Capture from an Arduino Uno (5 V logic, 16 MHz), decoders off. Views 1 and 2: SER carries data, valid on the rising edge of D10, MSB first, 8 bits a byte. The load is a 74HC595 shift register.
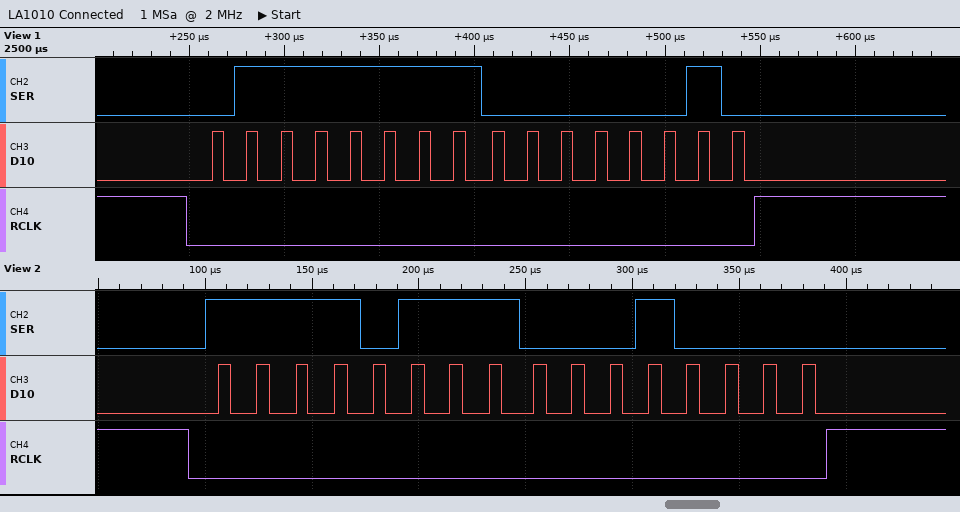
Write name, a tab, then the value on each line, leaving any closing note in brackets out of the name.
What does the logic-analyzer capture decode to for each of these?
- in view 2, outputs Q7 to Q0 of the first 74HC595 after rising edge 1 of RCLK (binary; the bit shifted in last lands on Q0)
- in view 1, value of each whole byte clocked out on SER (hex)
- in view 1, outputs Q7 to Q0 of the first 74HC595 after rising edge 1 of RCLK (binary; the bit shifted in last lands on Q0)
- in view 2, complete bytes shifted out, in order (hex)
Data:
in view 2, outputs Q7 to Q0 of the first 74HC595 after rising edge 1 of RCLK	00010000
in view 1, value of each whole byte clocked out on SER	7F 02
in view 1, outputs Q7 to Q0 of the first 74HC595 after rising edge 1 of RCLK	00000010
in view 2, complete bytes shifted out, in order	0xF7 0x10
